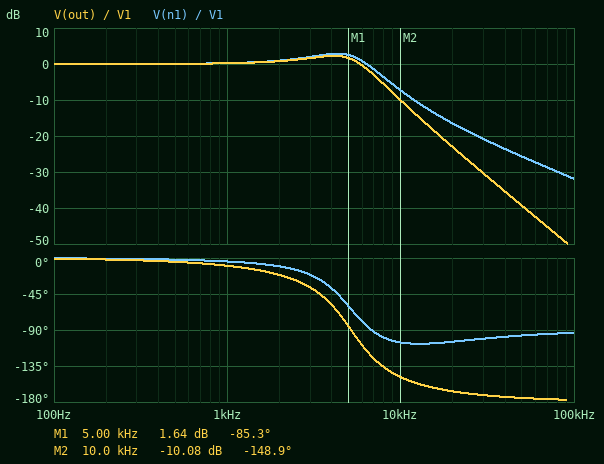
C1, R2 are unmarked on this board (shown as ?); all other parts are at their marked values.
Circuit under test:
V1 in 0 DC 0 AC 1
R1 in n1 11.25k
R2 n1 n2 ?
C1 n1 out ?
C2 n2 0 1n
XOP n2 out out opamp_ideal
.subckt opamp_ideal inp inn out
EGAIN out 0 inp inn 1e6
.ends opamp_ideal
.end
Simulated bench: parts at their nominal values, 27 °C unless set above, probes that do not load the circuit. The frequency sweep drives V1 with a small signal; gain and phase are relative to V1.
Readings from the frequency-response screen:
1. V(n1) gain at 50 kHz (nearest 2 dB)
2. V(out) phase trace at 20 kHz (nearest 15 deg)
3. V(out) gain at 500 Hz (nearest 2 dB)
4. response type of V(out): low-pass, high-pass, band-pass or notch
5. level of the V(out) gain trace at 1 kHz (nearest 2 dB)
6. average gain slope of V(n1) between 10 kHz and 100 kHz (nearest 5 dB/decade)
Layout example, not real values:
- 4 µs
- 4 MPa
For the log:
- -26 dB
- -165 deg
- 0 dB
- low-pass
- 0 dB
- -25 dB/decade
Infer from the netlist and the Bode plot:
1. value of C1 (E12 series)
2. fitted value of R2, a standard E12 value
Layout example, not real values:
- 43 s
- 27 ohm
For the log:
- 5.6 nF
- 15 kΩ
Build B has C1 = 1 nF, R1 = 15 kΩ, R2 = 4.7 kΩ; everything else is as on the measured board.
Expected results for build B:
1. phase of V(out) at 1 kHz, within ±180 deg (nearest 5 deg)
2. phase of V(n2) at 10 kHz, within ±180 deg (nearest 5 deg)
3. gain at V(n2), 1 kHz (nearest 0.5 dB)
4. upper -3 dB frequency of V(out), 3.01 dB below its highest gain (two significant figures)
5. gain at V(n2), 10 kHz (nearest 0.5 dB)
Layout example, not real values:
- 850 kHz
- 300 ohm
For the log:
- -5 deg
- -60 deg
- 0 dB
- 9.8 kHz
- -3.0 dB
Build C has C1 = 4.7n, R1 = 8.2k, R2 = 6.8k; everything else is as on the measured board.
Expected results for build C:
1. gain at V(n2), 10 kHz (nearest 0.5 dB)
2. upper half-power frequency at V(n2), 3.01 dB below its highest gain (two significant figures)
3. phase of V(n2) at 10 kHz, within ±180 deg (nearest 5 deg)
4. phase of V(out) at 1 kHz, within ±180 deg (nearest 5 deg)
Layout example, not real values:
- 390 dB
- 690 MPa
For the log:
- 0.5 dB
- 12 kHz
- -90 deg
- -5 deg
